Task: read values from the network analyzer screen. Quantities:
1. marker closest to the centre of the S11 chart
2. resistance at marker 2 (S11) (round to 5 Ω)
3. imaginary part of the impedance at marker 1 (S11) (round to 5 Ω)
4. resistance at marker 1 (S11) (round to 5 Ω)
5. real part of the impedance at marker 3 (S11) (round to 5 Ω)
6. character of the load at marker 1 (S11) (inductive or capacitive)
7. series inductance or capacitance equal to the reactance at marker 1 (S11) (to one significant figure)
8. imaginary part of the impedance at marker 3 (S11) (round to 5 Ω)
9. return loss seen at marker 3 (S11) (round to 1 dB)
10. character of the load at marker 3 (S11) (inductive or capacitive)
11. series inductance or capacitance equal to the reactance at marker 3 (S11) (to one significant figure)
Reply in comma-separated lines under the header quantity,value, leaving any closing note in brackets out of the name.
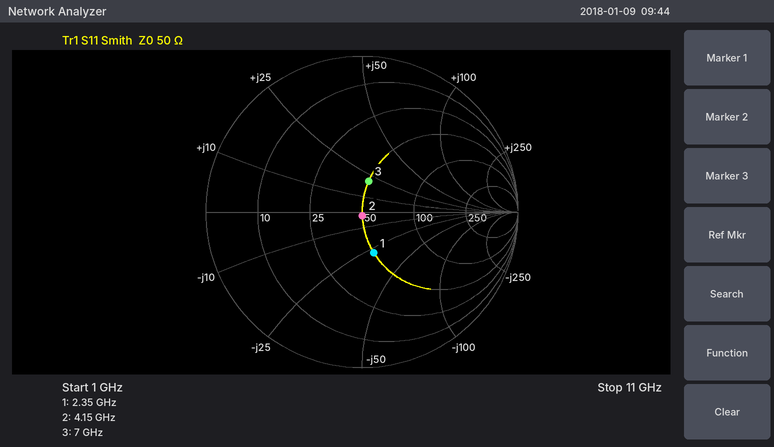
quantity,value
marker closest to the centre of the S11 chart,marker 2
resistance at marker 2 (S11),50 Ω
imaginary part of the impedance at marker 1 (S11),-30 Ω
resistance at marker 1 (S11),50 Ω
real part of the impedance at marker 3 (S11),50 Ω
character of the load at marker 1 (S11),capacitive
series inductance or capacitance equal to the reactance at marker 1 (S11),2 pF
imaginary part of the impedance at marker 3 (S11),+20 Ω
return loss seen at marker 3 (S11),14 dB
character of the load at marker 3 (S11),inductive
series inductance or capacitance equal to the reactance at marker 3 (S11),500 pH
